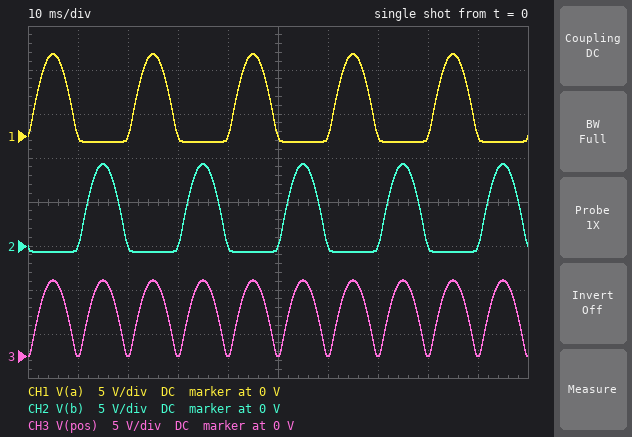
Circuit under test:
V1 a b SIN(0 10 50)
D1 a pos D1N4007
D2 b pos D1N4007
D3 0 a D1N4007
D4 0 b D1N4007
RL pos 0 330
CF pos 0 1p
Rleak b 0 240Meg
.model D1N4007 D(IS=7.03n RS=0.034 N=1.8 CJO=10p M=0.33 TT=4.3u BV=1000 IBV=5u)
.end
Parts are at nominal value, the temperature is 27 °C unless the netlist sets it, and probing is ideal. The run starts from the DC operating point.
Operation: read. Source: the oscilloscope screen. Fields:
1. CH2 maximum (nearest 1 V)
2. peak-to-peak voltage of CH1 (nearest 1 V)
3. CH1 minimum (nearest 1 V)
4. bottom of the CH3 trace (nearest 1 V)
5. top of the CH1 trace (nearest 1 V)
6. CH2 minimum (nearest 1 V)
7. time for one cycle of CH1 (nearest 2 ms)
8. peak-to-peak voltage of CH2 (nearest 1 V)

9 V
10 V
-1 V
0 V
9 V
-1 V
20 ms
10 V
